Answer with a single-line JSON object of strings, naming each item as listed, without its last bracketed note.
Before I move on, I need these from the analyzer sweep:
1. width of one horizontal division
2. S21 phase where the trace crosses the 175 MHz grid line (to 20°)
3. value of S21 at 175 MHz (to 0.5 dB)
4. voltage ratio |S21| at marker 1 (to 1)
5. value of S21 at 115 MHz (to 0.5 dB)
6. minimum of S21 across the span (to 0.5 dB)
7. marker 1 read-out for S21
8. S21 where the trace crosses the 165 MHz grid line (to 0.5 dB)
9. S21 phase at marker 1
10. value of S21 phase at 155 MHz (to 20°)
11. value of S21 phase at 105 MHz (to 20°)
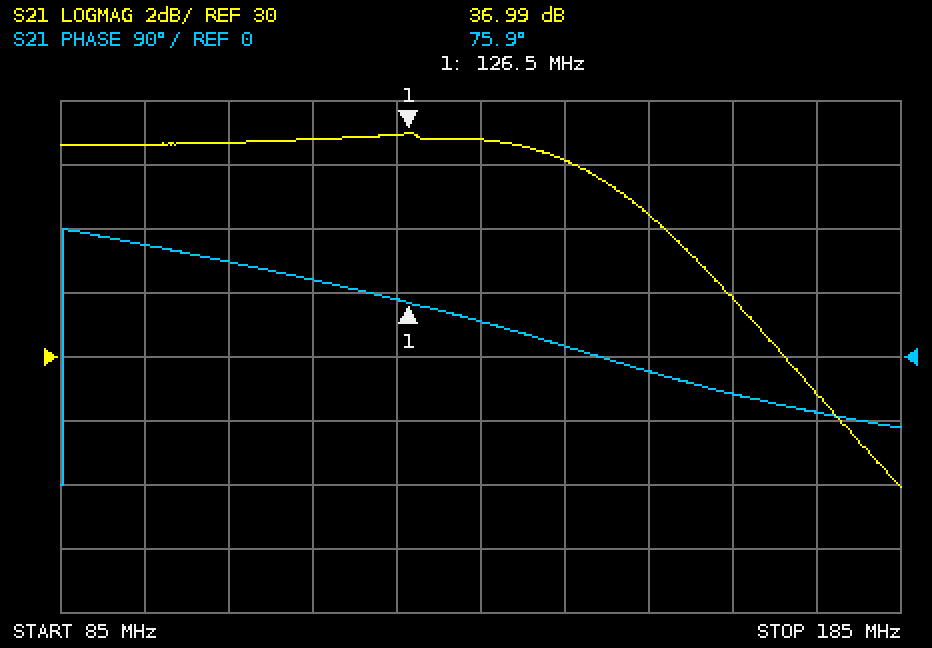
{"width of one horizontal division": "10 MHz", "S21 phase where the trace crosses the 175 MHz grid line": "-80°", "value of S21 at 175 MHz": "29.0 dB", "voltage ratio |S21| at marker 1": "71", "value of S21 at 115 MHz": "37.0 dB", "minimum of S21 across the span": "26.0 dB", "marker 1 read-out for S21": "36.99 dB", "S21 where the trace crosses the 165 MHz grid line": "32.0 dB", "S21 phase at marker 1": "75.9°", "value of S21 phase at 155 MHz": "-20°", "value of S21 phase at 105 MHz": "140°"}
